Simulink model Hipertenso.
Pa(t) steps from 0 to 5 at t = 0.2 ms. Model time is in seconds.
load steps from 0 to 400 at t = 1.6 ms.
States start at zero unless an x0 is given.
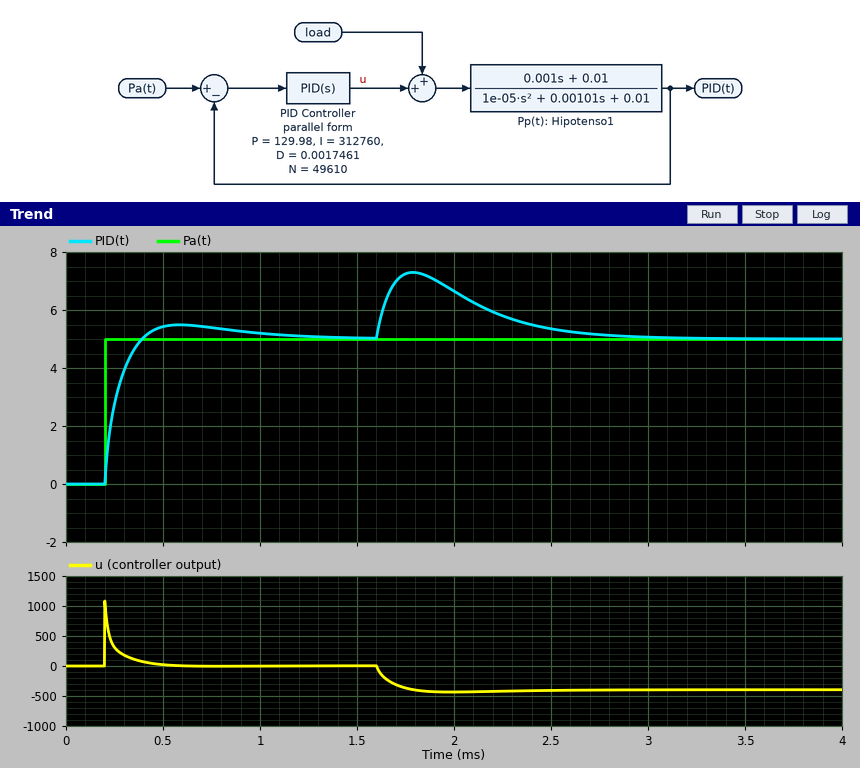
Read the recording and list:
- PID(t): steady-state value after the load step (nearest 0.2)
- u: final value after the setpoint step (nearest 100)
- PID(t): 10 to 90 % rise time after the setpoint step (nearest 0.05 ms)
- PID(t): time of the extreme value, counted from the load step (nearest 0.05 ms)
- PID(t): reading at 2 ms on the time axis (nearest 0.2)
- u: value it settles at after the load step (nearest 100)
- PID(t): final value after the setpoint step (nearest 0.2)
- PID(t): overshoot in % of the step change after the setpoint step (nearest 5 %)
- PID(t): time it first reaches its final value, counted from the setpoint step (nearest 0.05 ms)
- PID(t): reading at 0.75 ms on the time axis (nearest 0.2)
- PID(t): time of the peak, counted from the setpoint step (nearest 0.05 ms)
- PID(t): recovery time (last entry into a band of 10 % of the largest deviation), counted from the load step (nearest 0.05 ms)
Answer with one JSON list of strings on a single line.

["5.0", "0", "0.15 ms", "0.20 ms", "6.6", "-400", "5.0", "10 %", "0.20 ms", "5.4", "0.40 ms", "1.05 ms"]
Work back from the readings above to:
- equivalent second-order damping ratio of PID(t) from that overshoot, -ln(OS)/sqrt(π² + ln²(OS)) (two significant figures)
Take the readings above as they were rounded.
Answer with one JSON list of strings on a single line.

["0.59"]
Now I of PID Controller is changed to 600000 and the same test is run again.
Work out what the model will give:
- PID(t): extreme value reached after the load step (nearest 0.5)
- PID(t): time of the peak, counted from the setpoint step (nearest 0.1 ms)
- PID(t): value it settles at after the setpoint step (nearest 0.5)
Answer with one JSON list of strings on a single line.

["7.0", "0.3 ms", "5.0"]
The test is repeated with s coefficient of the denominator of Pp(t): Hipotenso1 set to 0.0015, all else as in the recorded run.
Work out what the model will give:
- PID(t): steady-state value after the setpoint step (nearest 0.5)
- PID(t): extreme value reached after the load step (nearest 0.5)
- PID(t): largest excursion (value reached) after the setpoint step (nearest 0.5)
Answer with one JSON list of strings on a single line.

["5.0", "7.5", "5.5"]
